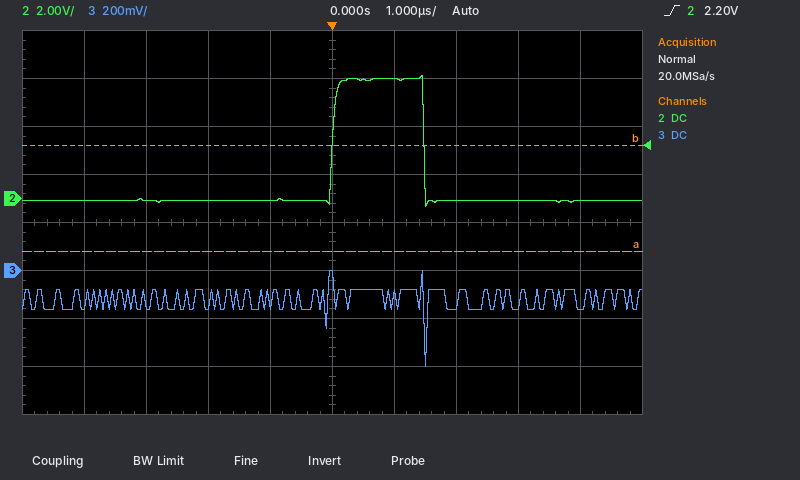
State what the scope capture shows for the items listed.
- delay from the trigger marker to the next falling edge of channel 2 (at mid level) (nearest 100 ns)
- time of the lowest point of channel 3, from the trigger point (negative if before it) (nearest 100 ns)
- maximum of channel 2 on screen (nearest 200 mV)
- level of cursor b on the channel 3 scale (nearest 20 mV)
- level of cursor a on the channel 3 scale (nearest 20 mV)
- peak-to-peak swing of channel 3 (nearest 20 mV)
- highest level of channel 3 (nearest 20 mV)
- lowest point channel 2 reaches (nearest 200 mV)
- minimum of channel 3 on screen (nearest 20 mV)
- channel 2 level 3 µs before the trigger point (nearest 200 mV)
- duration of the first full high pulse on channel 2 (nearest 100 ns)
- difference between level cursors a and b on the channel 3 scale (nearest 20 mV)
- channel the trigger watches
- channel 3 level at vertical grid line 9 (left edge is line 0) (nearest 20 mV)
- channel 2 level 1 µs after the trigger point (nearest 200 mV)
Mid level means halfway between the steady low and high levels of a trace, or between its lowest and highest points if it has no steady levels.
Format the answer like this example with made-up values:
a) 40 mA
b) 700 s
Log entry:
a) 1.5 µs
b) +1.5 µs
c) 5.2 V
d) 520 mV
e) 80 mV
f) 400 mV
g) 0 mV
h) -400 mV
i) -400 mV
j) 0.0 V
k) 1.5 µs
l) 440 mV
m) channel 2
n) -160 mV
o) 5.0 V
